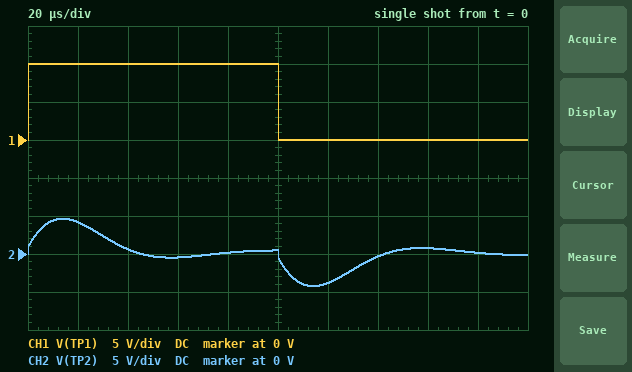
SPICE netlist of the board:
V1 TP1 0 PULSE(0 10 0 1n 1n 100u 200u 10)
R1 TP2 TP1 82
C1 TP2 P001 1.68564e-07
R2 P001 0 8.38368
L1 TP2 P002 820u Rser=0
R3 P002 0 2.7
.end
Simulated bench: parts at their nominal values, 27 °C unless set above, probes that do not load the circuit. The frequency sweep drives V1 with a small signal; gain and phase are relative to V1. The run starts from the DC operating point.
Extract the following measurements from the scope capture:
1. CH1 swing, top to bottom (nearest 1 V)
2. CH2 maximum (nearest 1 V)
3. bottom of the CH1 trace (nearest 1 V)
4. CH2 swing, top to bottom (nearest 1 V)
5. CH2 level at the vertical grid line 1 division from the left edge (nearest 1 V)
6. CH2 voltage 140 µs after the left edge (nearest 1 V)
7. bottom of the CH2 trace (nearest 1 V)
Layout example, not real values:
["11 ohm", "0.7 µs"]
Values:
["10 V", "5 V", "0 V", "9 V", "4 V", "0 V", "-4 V"]
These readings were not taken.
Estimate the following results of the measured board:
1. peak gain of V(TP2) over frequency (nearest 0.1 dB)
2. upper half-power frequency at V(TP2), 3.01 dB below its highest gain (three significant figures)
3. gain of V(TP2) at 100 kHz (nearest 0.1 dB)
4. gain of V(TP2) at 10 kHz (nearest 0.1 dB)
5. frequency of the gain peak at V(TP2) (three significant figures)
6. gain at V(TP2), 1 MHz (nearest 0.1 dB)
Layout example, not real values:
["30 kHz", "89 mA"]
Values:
["-1.5 dB", "20.9 kHz", "-17.0 dB", "-2.7 dB", "13.1 kHz", "-20.6 dB"]
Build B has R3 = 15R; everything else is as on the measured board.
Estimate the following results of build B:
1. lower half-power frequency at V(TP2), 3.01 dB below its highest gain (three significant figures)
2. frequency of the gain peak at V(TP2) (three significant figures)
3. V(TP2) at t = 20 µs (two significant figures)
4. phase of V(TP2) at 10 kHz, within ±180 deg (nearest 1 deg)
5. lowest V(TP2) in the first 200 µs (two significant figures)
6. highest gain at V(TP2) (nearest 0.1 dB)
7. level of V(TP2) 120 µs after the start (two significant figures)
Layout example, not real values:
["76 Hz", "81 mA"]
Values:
["8.19 kHz", "13.9 kHz", "4.5 V", "22 deg", "-3.2 V", "-2.8 dB", "-2.9 V"]
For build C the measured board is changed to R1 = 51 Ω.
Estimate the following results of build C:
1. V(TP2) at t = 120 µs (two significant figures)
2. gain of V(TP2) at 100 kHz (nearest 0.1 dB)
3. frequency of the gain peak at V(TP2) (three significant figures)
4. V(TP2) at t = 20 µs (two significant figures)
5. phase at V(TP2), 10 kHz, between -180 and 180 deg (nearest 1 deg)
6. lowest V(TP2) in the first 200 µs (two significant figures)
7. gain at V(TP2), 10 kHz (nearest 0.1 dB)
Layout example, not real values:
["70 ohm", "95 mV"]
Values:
["-4.7 V", "-13.4 dB", "12.9 kHz", "5.2 V", "22 deg", "-5.4 V", "-1.5 dB"]
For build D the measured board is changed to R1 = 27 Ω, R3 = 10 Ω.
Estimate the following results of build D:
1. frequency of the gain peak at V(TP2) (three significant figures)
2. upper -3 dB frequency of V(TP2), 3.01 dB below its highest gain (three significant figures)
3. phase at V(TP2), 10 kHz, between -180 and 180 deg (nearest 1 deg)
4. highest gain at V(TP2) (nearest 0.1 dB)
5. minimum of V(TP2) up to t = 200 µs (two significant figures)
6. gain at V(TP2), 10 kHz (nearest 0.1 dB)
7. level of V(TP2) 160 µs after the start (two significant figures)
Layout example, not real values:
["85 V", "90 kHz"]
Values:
["13.8 kHz", "37.2 kHz", "11 deg", "-0.8 dB", "-4.8 V", "-1.2 dB", "-500 mV"]
